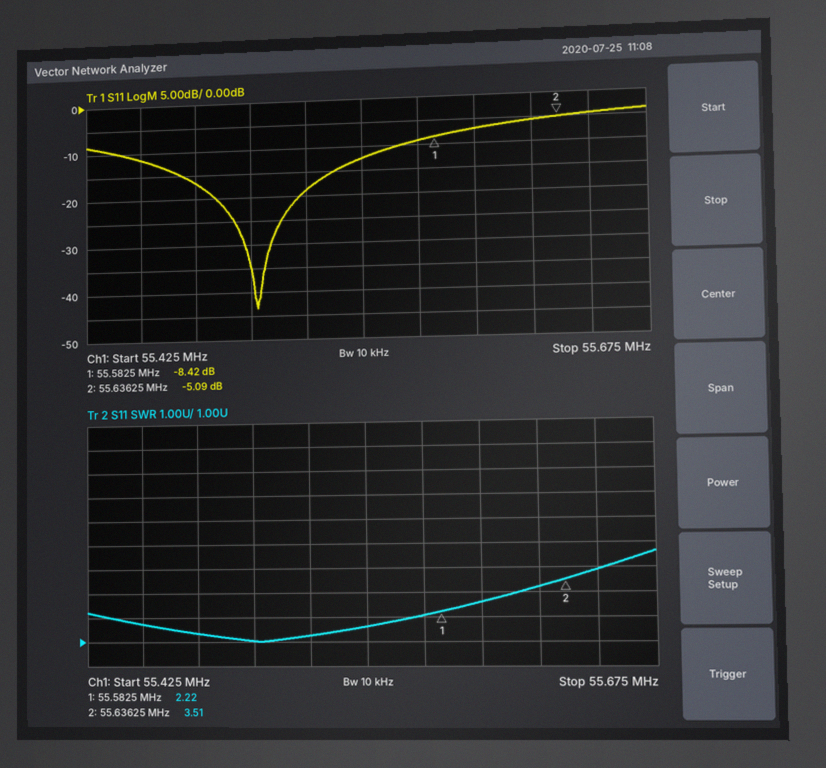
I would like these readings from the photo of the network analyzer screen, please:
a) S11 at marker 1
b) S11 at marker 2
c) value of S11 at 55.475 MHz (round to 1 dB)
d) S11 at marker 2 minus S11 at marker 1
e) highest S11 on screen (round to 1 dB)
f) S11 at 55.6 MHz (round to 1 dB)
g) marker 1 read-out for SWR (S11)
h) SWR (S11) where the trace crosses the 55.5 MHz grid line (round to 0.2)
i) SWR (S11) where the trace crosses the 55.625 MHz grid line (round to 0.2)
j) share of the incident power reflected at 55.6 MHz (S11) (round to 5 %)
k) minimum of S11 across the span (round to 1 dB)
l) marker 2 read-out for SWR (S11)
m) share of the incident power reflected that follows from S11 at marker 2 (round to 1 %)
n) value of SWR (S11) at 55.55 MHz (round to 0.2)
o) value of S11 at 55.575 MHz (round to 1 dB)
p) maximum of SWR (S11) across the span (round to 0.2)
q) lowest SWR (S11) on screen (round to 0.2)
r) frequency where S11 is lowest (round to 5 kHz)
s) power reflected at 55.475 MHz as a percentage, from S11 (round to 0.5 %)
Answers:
-8.42 dB
-5.09 dB
-17 dB
3.33 dB
-4 dB
-7 dB
2.22
1.0
3.2
20 %
-43 dB
3.51
31 %
1.6
-9 dB
4.6
1.0
55.505 MHz
2.0 %
